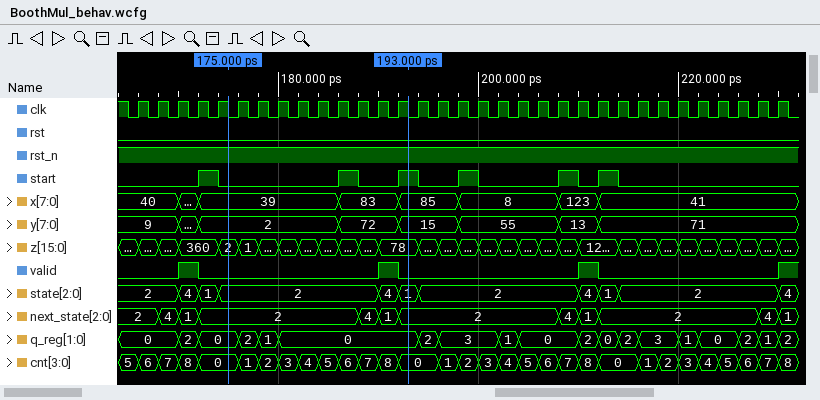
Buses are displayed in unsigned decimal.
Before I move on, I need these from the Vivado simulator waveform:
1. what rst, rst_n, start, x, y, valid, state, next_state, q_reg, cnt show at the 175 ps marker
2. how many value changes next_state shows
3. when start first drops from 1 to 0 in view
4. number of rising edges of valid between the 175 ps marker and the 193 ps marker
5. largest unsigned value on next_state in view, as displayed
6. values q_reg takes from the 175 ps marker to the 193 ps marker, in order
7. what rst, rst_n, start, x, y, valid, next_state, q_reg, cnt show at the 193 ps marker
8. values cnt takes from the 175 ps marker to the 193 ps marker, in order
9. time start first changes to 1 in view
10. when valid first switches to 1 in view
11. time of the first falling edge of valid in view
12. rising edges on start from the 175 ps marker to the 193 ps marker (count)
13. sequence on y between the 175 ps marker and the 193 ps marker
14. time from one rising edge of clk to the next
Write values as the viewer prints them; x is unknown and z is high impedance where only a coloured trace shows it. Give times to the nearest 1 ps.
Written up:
rst=0, rst_n=1, start=0, x=39, y=2, valid=0, state=2, next_state=2, q_reg=0, cnt=0
11
174 ps
1
4
0, 2, 1, 0
rst=0, rst_n=1, start=1, x=85, y=15, valid=0, next_state=2, q_reg=0, cnt=0
0, 1, 2, 3, 4, 5, 6, 7, 8, 0
172 ps
170 ps
172 ps
2
2, 72, 15
2 ps
